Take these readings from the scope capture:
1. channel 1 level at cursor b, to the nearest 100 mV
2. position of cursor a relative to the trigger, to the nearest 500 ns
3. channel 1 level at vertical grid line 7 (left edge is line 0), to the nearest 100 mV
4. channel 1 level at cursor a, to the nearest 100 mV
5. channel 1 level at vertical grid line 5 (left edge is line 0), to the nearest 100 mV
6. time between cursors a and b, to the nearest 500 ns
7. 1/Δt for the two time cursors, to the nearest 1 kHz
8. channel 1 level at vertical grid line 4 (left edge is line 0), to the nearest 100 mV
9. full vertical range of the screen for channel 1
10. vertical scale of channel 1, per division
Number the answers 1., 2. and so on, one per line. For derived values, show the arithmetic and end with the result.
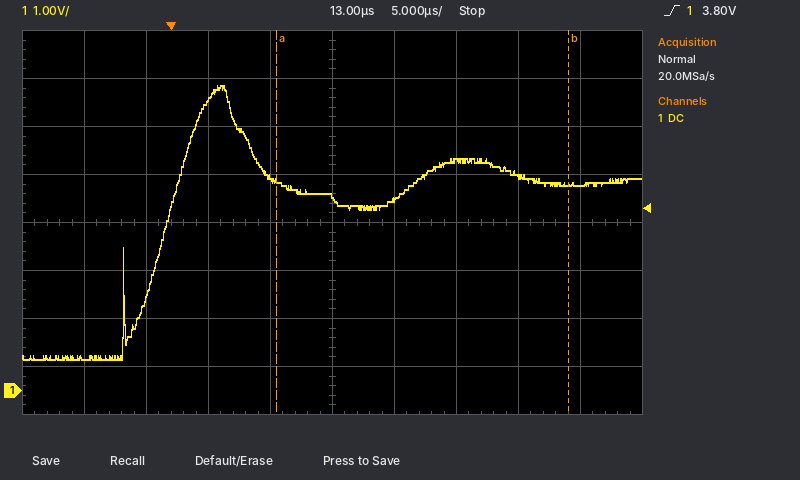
1. 4.3 V
2. +8.5 µs
3. 4.8 V
4. 4.4 V
5. 4.0 V
6. 23.5 µs
7. 1 / 23.5 µs ≈ 43 kHz
8. 4.4 V
9. 8 V
10. 1 V
